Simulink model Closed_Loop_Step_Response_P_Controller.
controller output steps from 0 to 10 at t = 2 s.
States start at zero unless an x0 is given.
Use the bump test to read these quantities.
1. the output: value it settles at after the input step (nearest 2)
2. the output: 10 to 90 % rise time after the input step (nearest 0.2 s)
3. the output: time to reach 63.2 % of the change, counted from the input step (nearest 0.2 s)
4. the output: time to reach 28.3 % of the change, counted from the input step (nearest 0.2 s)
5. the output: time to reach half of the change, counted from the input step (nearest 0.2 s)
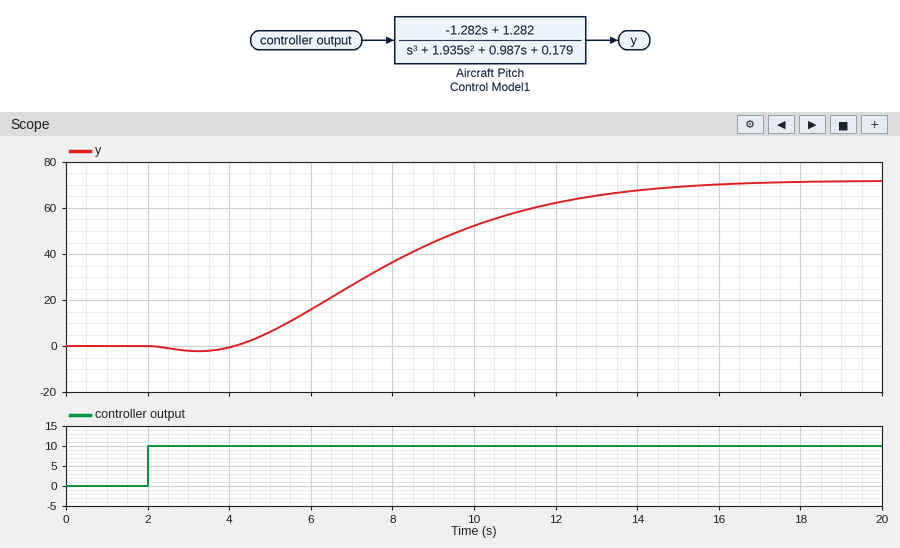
72
7.6 s
7.0 s
4.4 s
6.0 s
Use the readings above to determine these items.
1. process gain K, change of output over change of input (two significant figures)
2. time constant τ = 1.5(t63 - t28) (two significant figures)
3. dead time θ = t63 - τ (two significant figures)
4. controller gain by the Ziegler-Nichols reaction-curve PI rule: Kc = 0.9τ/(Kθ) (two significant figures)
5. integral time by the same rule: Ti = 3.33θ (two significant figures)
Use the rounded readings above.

7.2
3.9 s
3.1 s
0.16
10 s
